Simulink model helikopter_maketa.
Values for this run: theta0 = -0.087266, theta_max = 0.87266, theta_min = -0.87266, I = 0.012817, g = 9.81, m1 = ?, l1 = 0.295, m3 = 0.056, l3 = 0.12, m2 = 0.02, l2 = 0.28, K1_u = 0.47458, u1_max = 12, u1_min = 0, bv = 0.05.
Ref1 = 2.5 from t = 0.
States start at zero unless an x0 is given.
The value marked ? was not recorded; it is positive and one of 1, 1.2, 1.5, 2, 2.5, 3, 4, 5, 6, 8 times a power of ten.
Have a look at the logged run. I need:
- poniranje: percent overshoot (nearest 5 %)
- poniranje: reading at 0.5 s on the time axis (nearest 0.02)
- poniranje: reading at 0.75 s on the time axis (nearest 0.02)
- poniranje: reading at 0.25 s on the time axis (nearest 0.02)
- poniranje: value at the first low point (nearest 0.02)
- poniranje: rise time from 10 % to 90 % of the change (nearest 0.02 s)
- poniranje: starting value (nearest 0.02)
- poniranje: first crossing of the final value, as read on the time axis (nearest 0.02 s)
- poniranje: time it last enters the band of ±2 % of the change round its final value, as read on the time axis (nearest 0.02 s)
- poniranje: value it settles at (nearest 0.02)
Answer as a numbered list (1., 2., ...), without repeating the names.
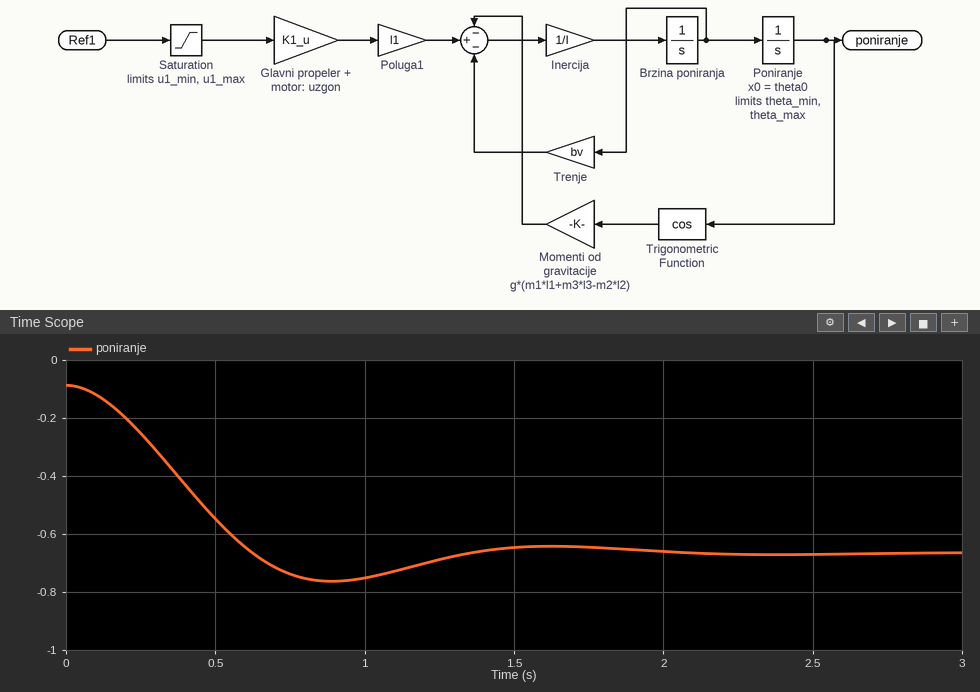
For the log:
1. 15 %
2. -0.54
3. -0.74
4. -0.26
5. -0.76
6. 0.42 s
7. -0.08
8. 0.62 s
9. 1.90 s
10. -0.66
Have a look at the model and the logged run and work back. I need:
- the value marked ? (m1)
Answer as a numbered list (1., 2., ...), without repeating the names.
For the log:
1. 0.15
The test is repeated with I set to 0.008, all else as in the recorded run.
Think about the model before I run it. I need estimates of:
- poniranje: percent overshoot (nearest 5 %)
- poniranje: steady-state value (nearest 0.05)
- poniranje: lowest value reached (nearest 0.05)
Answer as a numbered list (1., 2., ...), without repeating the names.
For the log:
1. 10 %
2. -0.65
3. -0.70
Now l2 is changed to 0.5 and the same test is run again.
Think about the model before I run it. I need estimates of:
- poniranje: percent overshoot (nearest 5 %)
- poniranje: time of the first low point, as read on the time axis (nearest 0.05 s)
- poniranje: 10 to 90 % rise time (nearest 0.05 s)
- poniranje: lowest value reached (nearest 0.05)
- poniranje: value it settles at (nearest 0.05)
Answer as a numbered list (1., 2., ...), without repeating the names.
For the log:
1. 10 %
2. 1.10 s
3. 0.55 s
4. -0.55
5. -0.50
